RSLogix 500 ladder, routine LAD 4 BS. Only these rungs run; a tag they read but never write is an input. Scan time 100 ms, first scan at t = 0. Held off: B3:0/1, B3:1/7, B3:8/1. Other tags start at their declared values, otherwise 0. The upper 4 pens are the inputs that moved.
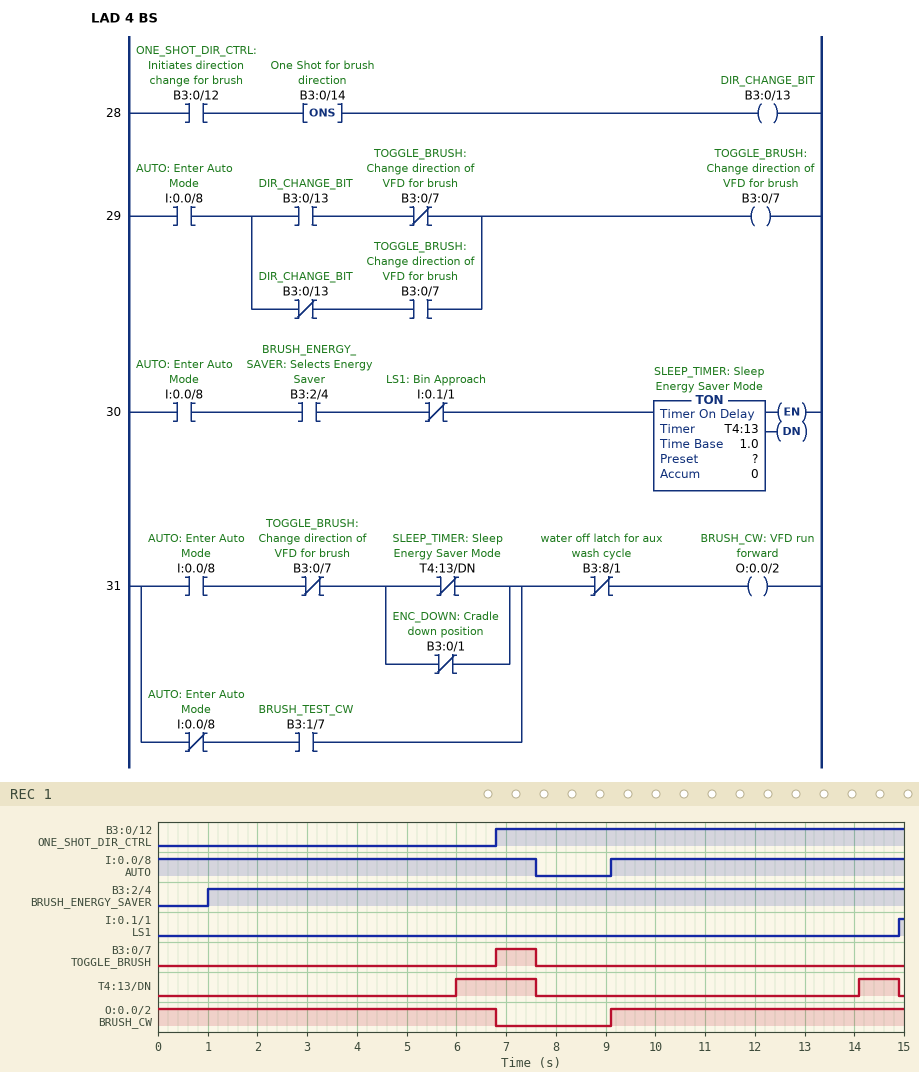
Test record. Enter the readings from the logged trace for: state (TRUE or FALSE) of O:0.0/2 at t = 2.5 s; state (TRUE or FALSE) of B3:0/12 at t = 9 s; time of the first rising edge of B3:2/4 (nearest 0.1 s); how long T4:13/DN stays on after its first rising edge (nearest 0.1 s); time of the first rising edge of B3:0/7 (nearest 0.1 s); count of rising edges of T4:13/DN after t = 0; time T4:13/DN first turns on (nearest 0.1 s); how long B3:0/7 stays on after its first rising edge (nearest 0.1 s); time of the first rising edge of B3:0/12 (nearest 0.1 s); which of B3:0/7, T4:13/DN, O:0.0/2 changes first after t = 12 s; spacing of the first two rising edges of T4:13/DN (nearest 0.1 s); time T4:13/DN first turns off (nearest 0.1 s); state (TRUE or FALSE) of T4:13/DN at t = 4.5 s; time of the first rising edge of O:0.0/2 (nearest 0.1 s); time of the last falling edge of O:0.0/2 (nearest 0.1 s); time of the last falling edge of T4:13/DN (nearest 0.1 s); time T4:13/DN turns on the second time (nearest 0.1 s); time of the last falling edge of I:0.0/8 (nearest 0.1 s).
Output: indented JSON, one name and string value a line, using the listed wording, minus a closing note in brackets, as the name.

{
  "state (TRUE or FALSE) of O:0.0/2 at t = 2.5 s": "TRUE",
  "state (TRUE or FALSE) of B3:0/12 at t = 9 s": "TRUE",
  "time of the first rising edge of B3:2/4": "1.0 s",
  "how long T4:13/DN stays on after its first rising edge": "1.6 s",
  "time of the first rising edge of B3:0/7": "6.8 s",
  "count of rising edges of T4:13/DN after t = 0": "2",
  "time T4:13/DN first turns on": "6.0 s",
  "how long B3:0/7 stays on after its first rising edge": "0.8 s",
  "time of the first rising edge of B3:0/12": "6.8 s",
  "which of B3:0/7, T4:13/DN, O:0.0/2 changes first after t = 12 s": "T4:13/DN",
  "spacing of the first two rising edges of T4:13/DN": "8.1 s",
  "time T4:13/DN first turns off": "7.6 s",
  "state (TRUE or FALSE) of T4:13/DN at t = 4.5 s": "FALSE",
  "time of the first rising edge of O:0.0/2": "9.1 s",
  "time of the last falling edge of O:0.0/2": "6.8 s",
  "time of the last falling edge of T4:13/DN": "14.9 s",
  "time T4:13/DN turns on the second time": "14.1 s",
  "time of the last falling edge of I:0.0/8": "7.6 s"
}
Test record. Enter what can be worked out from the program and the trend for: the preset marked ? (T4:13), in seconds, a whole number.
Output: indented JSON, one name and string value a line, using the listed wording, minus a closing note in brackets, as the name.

{
  "the preset marked ? (T4:13), in seconds, a whole number": "5 s"
}
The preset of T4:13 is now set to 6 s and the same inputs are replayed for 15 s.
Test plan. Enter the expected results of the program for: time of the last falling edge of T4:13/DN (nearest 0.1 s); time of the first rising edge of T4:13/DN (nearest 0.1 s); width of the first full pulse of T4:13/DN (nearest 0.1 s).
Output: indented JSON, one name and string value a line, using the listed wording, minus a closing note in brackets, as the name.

{
  "time of the last falling edge of T4:13/DN": "7.6 s",
  "time of the first rising edge of T4:13/DN": "7.0 s",
  "width of the first full pulse of T4:13/DN": "0.6 s"
}
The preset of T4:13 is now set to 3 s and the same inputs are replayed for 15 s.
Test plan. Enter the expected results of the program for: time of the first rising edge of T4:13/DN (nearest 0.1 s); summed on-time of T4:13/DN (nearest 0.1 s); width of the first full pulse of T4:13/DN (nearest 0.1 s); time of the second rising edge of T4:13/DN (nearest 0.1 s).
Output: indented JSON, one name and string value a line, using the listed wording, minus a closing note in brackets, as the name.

{
  "time of the first rising edge of T4:13/DN": "4.0 s",
  "summed on-time of T4:13/DN": "6.4 s",
  "width of the first full pulse of T4:13/DN": "3.6 s",
  "time of the second rising edge of T4:13/DN": "12.1 s"
}
